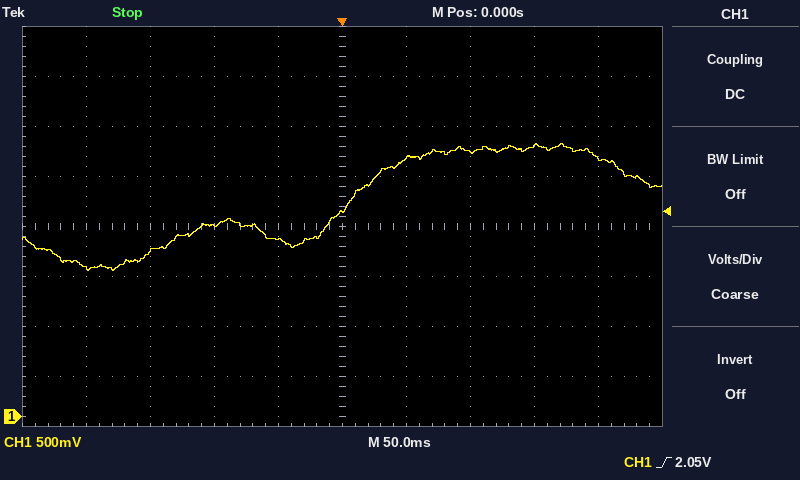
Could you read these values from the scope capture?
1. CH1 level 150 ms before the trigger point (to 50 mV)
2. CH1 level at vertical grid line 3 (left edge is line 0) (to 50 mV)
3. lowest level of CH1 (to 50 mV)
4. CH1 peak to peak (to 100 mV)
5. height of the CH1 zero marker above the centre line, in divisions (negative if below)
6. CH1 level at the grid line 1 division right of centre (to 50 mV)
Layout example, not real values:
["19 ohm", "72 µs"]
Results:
["1.65 V", "1.90 V", "1.45 V", "1.30 V", "-3.8 div", "2.60 V"]
